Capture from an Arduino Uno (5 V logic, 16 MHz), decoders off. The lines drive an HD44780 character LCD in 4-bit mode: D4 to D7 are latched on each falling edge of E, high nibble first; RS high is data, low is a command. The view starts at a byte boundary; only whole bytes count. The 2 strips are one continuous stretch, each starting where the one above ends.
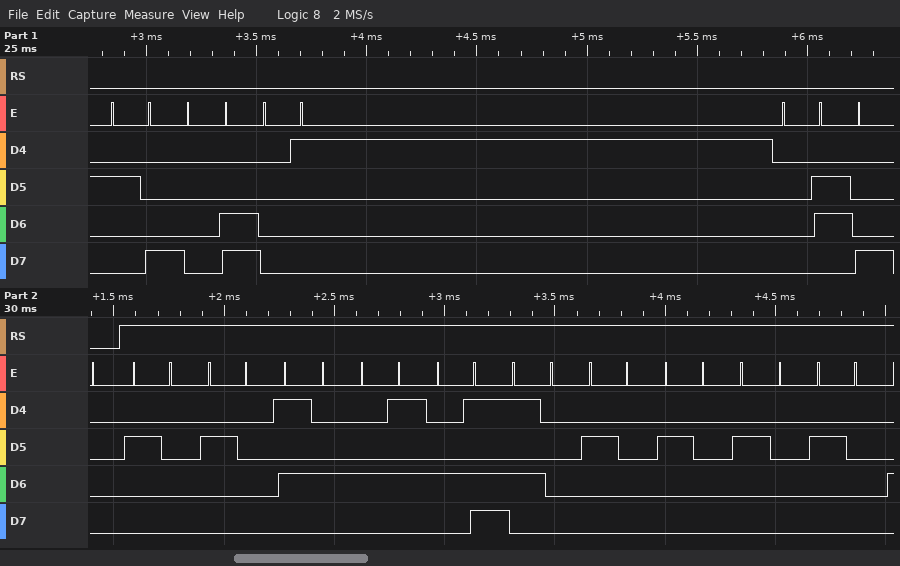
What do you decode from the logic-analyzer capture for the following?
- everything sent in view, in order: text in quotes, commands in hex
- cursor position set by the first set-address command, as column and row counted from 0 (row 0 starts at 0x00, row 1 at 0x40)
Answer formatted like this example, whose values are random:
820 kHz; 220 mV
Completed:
0x28 0x0C 0x01 0x06 0x80 "  TEMP    "; column 0, row 0
